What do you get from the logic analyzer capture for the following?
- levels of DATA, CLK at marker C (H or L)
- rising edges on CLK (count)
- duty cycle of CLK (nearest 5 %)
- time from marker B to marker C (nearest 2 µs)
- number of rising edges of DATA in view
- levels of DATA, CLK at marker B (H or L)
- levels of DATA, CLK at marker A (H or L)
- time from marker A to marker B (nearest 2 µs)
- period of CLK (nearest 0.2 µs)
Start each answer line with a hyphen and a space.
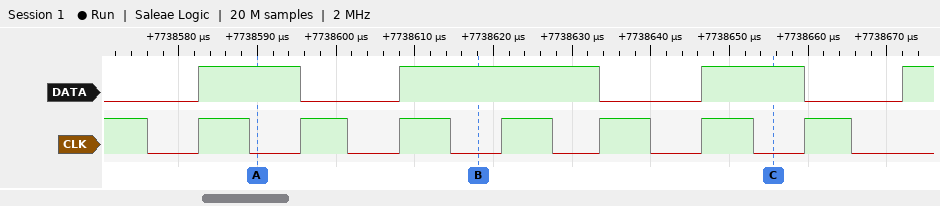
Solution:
- DATA=H, CLK=L
- 7
- 50 %
- 38 µs
- 4
- DATA=H, CLK=L
- DATA=H, CLK=L
- 28 µs
- 12.8 µs
